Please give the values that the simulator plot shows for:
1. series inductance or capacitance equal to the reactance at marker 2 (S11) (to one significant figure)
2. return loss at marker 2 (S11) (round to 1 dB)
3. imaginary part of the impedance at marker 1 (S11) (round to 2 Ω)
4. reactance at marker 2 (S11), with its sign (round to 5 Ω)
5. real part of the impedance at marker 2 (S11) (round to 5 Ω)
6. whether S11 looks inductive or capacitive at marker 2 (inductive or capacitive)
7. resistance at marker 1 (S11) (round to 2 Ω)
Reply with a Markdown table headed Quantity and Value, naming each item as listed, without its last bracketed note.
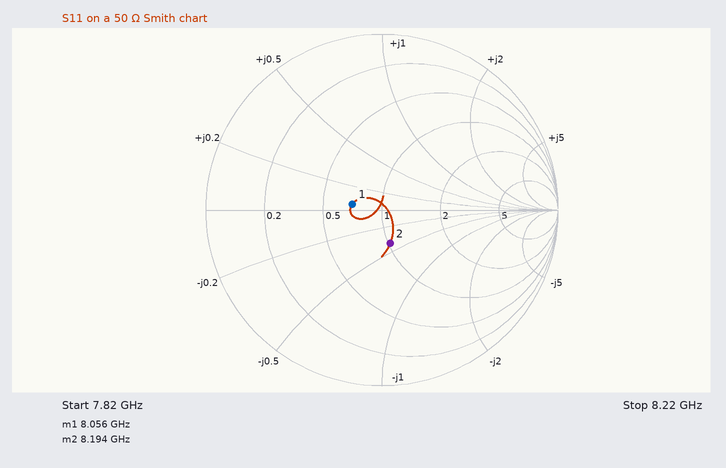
| Quantity | Value |
|---|---|
| series inductance or capacitance equal to the reactance at marker 2 (S11) | 1.0 pF |
| return loss at marker 2 (S11) | 14 dB |
| imaginary part of the impedance at marker 1 (S11) | +2 Ω |
| reactance at marker 2 (S11), with its sign | -20 Ω |
| real part of the impedance at marker 2 (S11) | 50 Ω |
| whether S11 looks inductive or capacitive at marker 2 | capacitive |
| resistance at marker 1 (S11) | 36 Ω |
